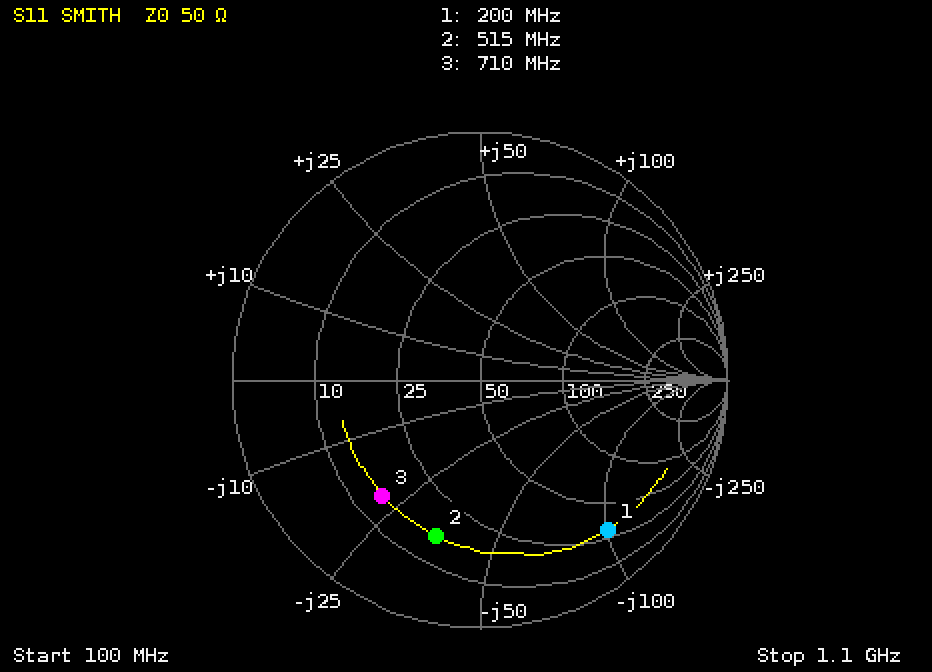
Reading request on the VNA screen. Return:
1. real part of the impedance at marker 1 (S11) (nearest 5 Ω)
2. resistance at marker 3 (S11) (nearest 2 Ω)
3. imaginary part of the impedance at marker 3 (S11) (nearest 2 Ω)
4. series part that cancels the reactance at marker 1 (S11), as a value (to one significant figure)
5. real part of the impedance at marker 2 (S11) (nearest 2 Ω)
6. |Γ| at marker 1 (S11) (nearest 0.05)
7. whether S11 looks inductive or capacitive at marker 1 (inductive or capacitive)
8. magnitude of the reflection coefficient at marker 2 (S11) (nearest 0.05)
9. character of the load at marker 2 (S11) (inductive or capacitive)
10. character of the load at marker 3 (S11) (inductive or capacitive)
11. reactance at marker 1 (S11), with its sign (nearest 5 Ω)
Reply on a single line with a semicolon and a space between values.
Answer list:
30 Ω; 14 Ω; -22 Ω; 80 nH; 16 Ω; 0.80; capacitive; 0.65; capacitive; capacitive; -100 Ω
